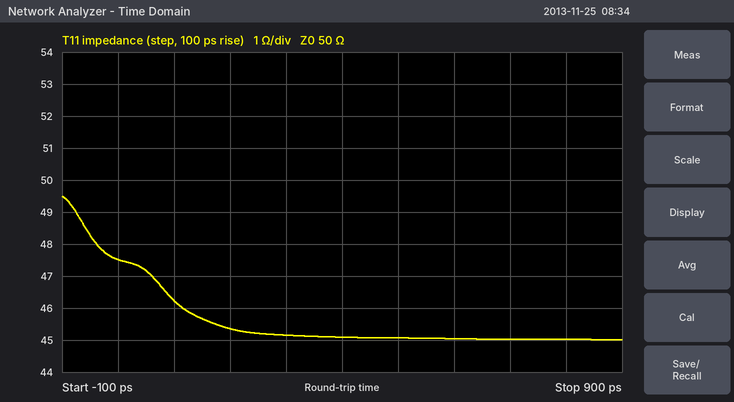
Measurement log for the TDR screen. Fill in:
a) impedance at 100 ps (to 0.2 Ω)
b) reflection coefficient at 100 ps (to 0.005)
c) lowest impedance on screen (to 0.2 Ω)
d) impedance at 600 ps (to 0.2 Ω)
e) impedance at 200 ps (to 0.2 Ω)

46.2 Ω
-0.040
45.0 Ω
45.0 Ω
45.4 Ω
